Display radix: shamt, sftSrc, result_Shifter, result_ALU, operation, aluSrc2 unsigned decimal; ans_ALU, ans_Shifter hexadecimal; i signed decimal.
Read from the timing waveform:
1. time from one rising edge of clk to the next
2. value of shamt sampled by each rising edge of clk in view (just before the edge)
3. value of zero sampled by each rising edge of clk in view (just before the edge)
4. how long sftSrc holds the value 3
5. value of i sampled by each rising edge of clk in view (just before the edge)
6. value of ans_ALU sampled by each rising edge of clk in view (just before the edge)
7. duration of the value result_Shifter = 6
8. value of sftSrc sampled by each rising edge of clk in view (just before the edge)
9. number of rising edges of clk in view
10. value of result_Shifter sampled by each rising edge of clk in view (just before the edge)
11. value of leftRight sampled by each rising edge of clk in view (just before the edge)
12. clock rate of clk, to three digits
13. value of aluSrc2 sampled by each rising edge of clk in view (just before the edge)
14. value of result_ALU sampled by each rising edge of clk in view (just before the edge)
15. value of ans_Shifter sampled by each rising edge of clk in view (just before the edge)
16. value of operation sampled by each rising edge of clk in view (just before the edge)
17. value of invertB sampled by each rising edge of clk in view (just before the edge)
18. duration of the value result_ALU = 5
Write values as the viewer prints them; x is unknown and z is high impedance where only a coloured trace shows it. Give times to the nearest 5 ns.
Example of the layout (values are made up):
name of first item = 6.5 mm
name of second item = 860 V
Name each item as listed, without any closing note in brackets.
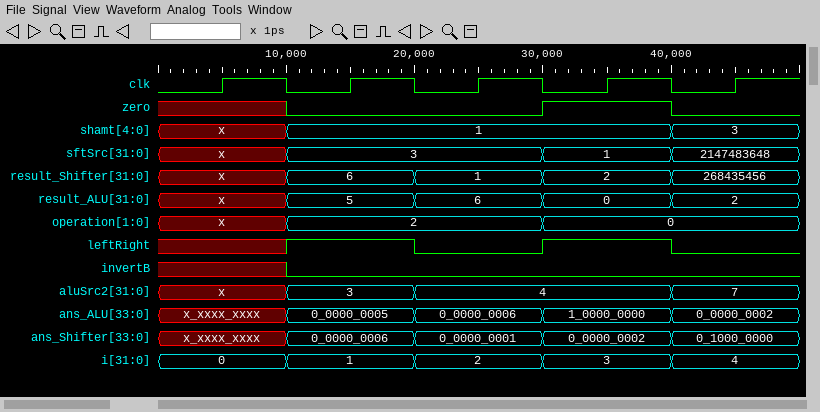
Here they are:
time from one rising edge of clk to the next = 10 ns
value of shamt sampled by each rising edge of clk in view = x, 1, 1, 1, 3
value of zero sampled by each rising edge of clk in view = x 0 0 1 0
how long sftSrc holds the value 3 = 20 ns
value of i sampled by each rising edge of clk in view = 0, 1, 2, 3, 4
value of ans_ALU sampled by each rising edge of clk in view = x_xxxx_xxxx, 0_0000_0005, 0_0000_0006, 1_0000_0000, 0_0000_0002
duration of the value result_Shifter = 6 = 10 ns
value of sftSrc sampled by each rising edge of clk in view = x, 3, 3, 1, 2147483648
number of rising edges of clk in view = 5
value of result_Shifter sampled by each rising edge of clk in view = x, 6, 1, 2, 268435456
value of leftRight sampled by each rising edge of clk in view = x 1 0 1 0
clock rate of clk, to three digits = 100 MHz
value of aluSrc2 sampled by each rising edge of clk in view = x, 3, 4, 4, 7
value of result_ALU sampled by each rising edge of clk in view = x, 5, 6, 0, 2
value of ans_Shifter sampled by each rising edge of clk in view = x_xxxx_xxxx, 0_0000_0006, 0_0000_0001, 0_0000_0002, 0_1000_0000
value of operation sampled by each rising edge of clk in view = x, 2, 2, 0, 0
value of invertB sampled by each rising edge of clk in view = x 0 0 0 0
duration of the value result_ALU = 5 = 10 ns
